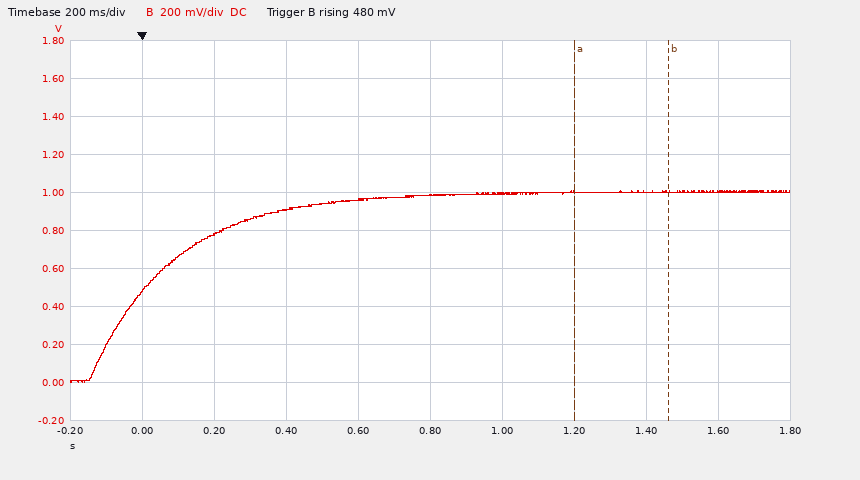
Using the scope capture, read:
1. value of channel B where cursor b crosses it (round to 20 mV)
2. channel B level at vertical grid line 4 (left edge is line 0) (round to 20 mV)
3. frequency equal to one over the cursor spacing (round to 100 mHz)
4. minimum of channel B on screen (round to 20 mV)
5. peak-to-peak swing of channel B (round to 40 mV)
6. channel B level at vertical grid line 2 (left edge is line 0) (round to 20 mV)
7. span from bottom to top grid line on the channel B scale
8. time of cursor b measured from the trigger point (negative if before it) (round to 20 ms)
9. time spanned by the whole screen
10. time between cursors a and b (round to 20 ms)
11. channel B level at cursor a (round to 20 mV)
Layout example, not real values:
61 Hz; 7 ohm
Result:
1.00 V; 960 mV; 3.8 Hz; 0 mV; 1.00 V; 780 mV; 2 V; +1.46 s; 2 s; 260 ms; 1.00 V
